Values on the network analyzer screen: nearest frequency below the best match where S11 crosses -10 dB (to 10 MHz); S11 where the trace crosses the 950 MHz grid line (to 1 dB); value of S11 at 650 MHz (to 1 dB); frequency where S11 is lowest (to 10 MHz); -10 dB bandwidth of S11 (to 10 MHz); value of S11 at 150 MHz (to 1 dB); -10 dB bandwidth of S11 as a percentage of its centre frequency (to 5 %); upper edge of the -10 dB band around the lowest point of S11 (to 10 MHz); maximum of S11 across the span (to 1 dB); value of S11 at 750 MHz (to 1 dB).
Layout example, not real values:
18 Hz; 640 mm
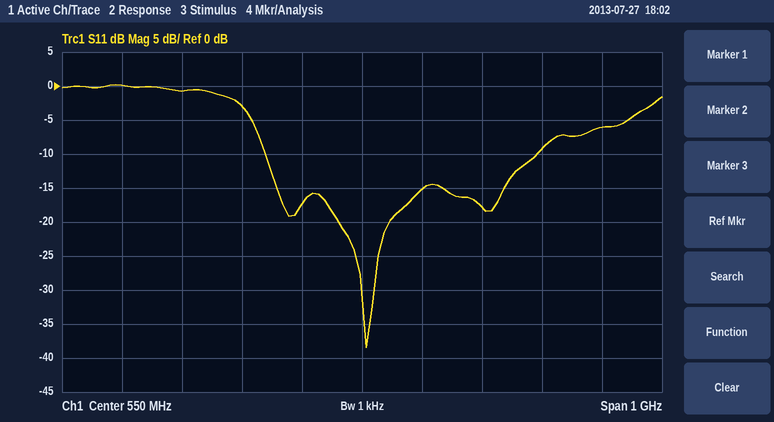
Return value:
390 MHz; -6 dB; -15 dB; 560 MHz; 450 MHz; 0 dB; 75 %; 840 MHz; 0 dB; -18 dB
